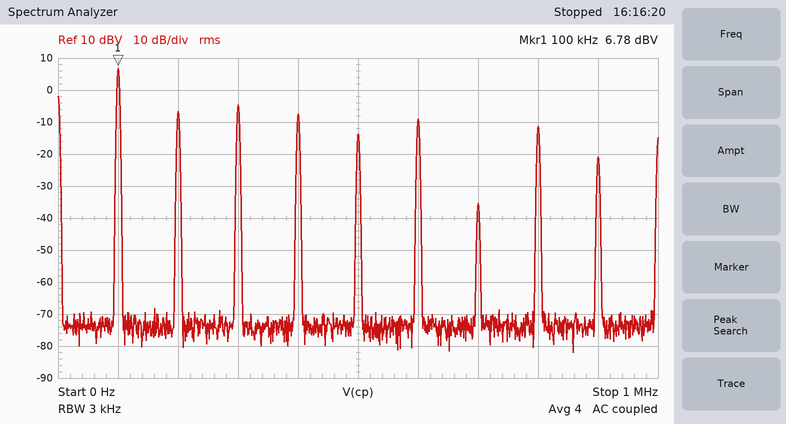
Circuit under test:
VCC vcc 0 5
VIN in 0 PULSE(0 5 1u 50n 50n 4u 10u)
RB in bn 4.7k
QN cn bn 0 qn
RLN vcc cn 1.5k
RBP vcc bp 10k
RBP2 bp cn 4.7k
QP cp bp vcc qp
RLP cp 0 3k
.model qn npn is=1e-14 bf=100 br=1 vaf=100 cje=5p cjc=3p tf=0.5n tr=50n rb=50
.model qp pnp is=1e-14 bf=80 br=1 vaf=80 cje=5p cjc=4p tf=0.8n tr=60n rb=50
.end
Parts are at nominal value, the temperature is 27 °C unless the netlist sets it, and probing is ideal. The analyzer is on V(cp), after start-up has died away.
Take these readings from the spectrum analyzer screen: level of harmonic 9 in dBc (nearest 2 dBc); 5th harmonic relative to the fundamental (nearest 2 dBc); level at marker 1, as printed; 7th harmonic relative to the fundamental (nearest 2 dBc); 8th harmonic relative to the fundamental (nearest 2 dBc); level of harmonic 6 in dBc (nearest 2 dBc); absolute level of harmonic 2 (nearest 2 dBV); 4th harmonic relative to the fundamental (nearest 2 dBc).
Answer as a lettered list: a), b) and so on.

a) -28 dBc
b) -20 dBc
c) 6.78 dBV
d) -42 dBc
e) -18 dBc
f) -16 dBc
g) -6 dBV
h) -14 dBc
